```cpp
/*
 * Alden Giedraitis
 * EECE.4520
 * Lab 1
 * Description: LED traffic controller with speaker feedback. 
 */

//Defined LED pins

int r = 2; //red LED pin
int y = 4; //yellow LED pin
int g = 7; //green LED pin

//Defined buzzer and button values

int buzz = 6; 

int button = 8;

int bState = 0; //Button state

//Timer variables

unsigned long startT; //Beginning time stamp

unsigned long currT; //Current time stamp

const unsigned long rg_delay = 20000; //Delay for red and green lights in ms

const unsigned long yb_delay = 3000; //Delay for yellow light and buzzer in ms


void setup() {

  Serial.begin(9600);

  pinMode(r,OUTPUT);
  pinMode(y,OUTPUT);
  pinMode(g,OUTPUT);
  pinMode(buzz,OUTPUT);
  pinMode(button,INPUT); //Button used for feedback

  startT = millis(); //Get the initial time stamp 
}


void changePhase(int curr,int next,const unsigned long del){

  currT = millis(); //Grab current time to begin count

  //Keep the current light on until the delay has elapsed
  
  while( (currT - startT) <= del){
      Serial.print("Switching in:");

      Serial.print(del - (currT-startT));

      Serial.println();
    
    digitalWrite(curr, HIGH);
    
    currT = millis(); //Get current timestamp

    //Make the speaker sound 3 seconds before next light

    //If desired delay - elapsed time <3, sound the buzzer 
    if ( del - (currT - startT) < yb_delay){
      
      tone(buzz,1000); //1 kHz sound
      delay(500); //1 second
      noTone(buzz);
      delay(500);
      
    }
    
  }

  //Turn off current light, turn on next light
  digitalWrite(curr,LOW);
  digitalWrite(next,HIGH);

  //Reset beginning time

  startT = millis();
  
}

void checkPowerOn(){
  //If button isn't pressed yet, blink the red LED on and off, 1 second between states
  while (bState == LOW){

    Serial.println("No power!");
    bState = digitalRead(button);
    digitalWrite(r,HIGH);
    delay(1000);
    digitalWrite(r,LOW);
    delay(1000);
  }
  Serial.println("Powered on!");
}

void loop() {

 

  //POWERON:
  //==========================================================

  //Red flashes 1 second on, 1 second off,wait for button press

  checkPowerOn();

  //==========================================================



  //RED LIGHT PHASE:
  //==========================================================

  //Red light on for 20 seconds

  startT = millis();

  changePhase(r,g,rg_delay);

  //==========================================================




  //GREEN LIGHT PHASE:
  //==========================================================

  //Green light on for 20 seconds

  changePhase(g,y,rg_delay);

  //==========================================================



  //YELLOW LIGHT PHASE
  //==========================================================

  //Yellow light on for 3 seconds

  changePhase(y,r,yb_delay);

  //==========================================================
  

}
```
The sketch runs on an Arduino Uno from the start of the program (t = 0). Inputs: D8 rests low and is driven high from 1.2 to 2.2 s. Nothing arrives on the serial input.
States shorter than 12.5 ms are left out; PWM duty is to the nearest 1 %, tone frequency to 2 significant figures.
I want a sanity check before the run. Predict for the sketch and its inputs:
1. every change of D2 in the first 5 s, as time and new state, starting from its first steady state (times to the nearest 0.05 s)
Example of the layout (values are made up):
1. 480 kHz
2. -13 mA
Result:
1. 0 s high; 1 s low; 2 s high; 3 s low; 4 s high
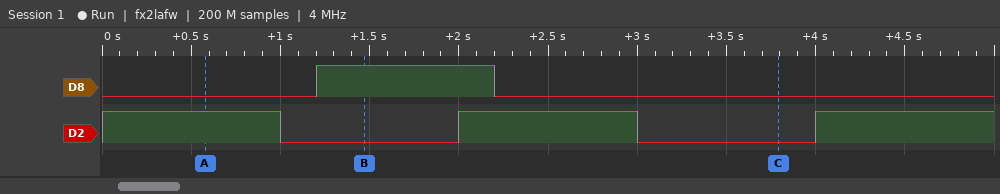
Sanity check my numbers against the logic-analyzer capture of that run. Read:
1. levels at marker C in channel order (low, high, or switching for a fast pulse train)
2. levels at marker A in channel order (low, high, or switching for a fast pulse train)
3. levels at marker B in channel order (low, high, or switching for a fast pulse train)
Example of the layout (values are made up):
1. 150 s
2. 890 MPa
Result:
1. D8 low, D2 low
2. D8 low, D2 high
3. D8 high, D2 low
